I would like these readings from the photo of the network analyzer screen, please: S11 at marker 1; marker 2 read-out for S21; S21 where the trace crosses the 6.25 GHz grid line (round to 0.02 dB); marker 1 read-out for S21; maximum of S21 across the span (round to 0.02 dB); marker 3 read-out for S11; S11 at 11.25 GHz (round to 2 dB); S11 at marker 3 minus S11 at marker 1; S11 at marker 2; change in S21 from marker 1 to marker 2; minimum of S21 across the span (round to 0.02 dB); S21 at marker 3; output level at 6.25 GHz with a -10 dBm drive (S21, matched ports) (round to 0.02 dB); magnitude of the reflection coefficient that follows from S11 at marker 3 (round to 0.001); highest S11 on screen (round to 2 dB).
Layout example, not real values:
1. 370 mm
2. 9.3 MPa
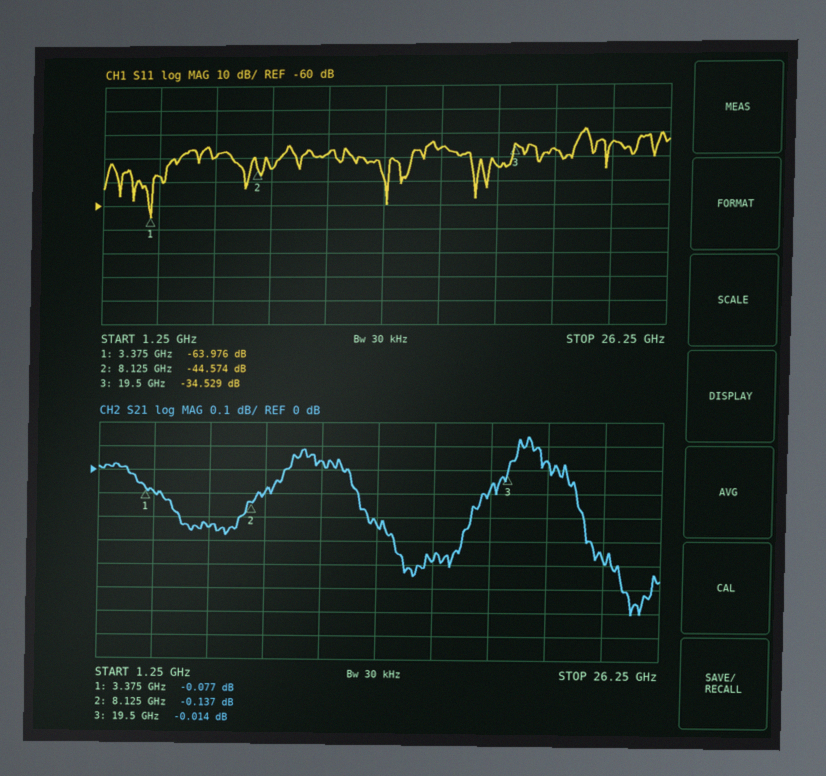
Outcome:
1. -63.976 dB
2. -0.137 dB
3. -0.24 dB
4. -0.077 dB
5. 0.14 dB
6. -34.529 dB
7. -38 dB
8. 29.447 dB
9. -44.574 dB
10. -0.060 dB
11. -0.60 dB
12. -0.014 dB
13. -10.24 dBm
14. 0.019
15. -28 dB
